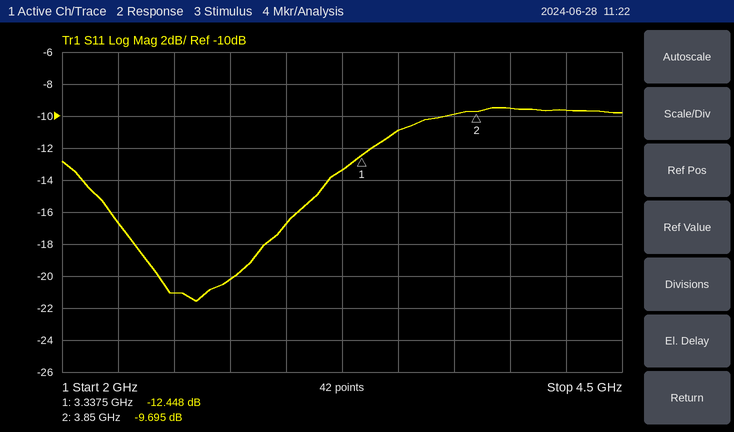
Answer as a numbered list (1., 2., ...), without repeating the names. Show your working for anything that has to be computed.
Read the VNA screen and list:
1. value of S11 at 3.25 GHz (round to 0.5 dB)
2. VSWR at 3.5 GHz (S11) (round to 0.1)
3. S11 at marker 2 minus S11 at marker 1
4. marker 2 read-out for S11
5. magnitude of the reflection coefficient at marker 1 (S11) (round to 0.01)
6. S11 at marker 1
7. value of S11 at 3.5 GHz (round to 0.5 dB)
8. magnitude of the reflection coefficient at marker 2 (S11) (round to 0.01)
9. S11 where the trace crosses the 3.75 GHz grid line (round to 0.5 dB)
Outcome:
1. -13.5 dB
2. |Γ| = 10^(-11/20) = 0.2818; VSWR = (1 + 0.2818)/(1 − 0.2818) ≈ 1.8
3. -9.695 − (-12.448) = 2.753 dB
4. -9.695 dB
5. 10^(-12.448/20) ≈ 0.24
6. -12.448 dB
7. -11.0 dB
8. 10^(-9.695/20) ≈ 0.33
9. -10.0 dB
